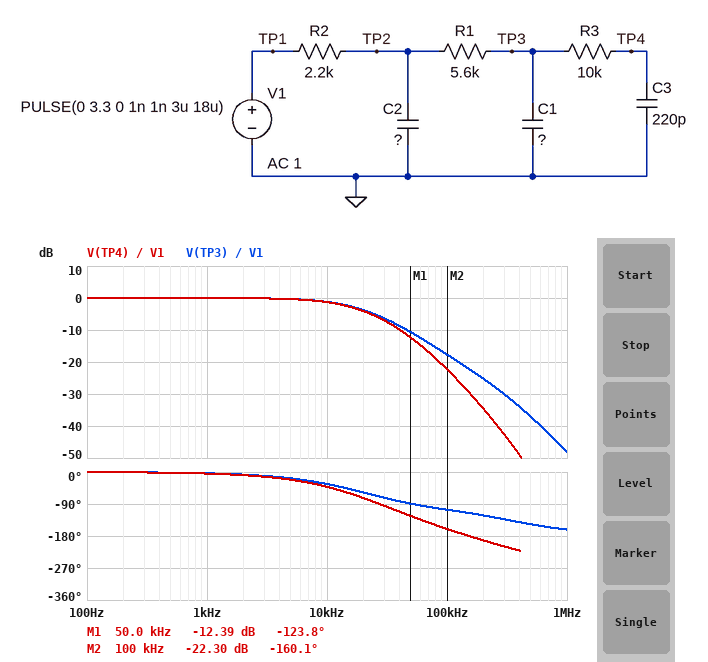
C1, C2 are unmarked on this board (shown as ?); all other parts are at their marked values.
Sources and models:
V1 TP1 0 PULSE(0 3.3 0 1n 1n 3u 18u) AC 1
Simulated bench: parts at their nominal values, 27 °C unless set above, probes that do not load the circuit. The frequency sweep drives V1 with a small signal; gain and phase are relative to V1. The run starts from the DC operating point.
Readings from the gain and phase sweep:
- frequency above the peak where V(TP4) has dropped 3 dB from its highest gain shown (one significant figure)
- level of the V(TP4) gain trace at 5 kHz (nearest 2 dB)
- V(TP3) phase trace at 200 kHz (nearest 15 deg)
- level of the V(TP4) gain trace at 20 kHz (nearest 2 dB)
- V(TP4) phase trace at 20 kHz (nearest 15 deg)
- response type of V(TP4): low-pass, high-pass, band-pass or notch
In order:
20 kHz
0 dB
-120 deg
-4 dB
-75 deg
low-pass
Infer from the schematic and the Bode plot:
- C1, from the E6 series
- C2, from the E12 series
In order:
150 pF
3.3 nF
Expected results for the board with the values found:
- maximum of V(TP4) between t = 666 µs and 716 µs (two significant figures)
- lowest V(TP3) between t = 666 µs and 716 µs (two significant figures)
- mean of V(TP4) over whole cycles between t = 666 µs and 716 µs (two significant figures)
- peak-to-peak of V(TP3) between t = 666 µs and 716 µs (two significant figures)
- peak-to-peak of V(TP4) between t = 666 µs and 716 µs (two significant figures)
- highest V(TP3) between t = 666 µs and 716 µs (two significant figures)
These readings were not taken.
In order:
770 mV
240 mV
550 mV
660 mV
470 mV
900 mV
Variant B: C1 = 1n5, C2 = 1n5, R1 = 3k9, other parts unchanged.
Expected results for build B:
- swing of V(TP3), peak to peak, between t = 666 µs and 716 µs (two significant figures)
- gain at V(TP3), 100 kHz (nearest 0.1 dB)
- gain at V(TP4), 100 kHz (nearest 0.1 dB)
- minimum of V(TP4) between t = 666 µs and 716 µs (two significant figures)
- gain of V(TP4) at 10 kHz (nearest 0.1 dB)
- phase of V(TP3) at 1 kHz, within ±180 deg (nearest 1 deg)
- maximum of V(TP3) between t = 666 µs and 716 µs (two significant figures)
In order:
480 mV
-20.7 dB
-25.4 dB
360 mV
-2.1 dB
-5 deg
790 mV
